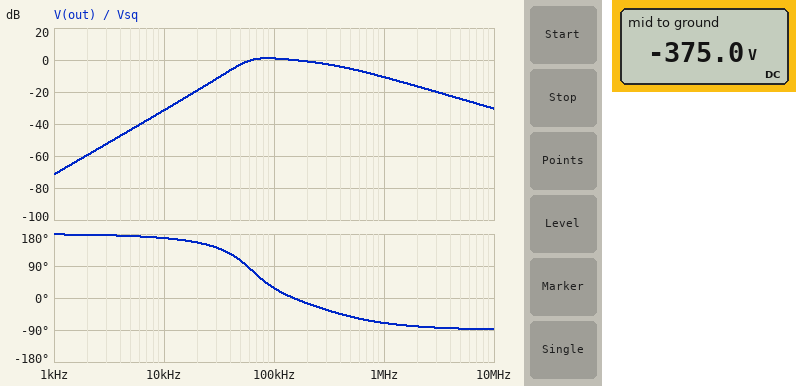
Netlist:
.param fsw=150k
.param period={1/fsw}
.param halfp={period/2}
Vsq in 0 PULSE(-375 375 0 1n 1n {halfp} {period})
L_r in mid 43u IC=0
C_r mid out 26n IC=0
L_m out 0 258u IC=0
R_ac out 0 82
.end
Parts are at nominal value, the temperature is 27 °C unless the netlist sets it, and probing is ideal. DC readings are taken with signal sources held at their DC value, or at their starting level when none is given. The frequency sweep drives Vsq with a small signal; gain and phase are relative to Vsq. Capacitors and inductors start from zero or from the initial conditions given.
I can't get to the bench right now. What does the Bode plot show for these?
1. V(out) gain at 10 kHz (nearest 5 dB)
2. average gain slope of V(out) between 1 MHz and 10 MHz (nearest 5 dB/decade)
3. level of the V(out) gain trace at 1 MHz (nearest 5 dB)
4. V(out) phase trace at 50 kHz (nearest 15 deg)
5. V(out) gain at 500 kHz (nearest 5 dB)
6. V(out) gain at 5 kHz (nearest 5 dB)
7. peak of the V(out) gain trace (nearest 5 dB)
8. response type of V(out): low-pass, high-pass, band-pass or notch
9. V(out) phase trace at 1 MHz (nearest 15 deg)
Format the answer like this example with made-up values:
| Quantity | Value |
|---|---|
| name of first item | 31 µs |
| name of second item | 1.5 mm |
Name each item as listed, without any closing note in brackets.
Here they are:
| Quantity | Value |
|---|---|
| V(out) gain at 10 kHz | -30 dB |
| average gain slope of V(out) between 1 MHz and 10 MHz | -20 dB/decade |
| level of the V(out) gain trace at 1 MHz | -10 dB |
| V(out) phase trace at 50 kHz | 105 deg |
| V(out) gain at 500 kHz | -5 dB |
| V(out) gain at 5 kHz | -45 dB |
| peak of the V(out) gain trace | 0 dB |
| response type of V(out): low-pass, high-pass, band-pass or notch | band-pass |
| V(out) phase trace at 1 MHz | -75 deg |
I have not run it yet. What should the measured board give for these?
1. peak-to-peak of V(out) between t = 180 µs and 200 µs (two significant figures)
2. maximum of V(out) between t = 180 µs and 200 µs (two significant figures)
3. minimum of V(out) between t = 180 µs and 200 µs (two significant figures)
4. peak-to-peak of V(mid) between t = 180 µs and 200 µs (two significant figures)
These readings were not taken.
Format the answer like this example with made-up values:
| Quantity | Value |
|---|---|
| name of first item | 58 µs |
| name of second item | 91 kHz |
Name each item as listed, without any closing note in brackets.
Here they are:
| Quantity | Value |
|---|---|
| peak-to-peak of V(out) between t = 180 µs and 200 µs | 920 V |
| maximum of V(out) between t = 180 µs and 200 µs | 460 V |
| minimum of V(out) between t = 180 µs and 200 µs | -460 V |
| peak-to-peak of V(mid) between t = 180 µs and 200 µs | 850 V |
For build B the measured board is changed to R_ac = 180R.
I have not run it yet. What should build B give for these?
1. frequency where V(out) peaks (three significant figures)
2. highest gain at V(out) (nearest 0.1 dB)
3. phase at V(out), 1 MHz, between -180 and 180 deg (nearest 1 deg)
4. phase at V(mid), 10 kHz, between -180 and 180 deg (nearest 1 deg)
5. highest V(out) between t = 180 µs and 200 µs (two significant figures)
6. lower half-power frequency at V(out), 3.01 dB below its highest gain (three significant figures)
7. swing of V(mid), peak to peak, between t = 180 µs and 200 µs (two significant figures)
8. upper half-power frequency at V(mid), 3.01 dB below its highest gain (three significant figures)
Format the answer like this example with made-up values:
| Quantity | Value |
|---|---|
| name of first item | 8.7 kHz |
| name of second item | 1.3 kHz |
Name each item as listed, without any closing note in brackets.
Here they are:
| Quantity | Value |
|---|---|
| frequency where V(out) peaks | 60.9 kHz |
| highest gain at V(out) | 6.2 dB |
| phase at V(out), 1 MHz, between -180 and 180 deg | -52 deg |
| phase at V(mid), 10 kHz, between -180 and 180 deg | 0 deg |
| highest V(out) between t = 180 µs and 200 µs | 430 V |
| lower half-power frequency at V(out), 3.01 dB below its highest gain | 50.1 kHz |
| swing of V(mid), peak to peak, between t = 180 µs and 200 µs | 720 V |
| upper half-power frequency at V(mid), 3.01 dB below its highest gain | 101 kHz |
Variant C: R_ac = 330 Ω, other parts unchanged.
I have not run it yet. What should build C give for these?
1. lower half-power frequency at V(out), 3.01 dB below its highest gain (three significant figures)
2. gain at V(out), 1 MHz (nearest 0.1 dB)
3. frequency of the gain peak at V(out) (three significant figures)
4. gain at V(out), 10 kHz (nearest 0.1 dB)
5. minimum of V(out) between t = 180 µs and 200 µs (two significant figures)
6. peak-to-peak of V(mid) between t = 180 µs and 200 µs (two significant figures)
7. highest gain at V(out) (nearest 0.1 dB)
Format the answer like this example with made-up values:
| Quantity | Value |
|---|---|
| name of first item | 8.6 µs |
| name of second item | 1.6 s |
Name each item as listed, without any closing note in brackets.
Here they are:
| Quantity | Value |
|---|---|
| lower half-power frequency at V(out), 3.01 dB below its highest gain | 52.0 kHz |
| gain at V(out), 1 MHz | -3.0 dB |
| frequency of the gain peak at V(out) | 58.0 kHz |
| gain at V(out), 10 kHz | -31.3 dB |
| minimum of V(out) between t = 180 µs and 200 µs | -400 V |
| peak-to-peak of V(mid) between t = 180 µs and 200 µs | 680 V |
| highest gain at V(out) | 11.2 dB |
